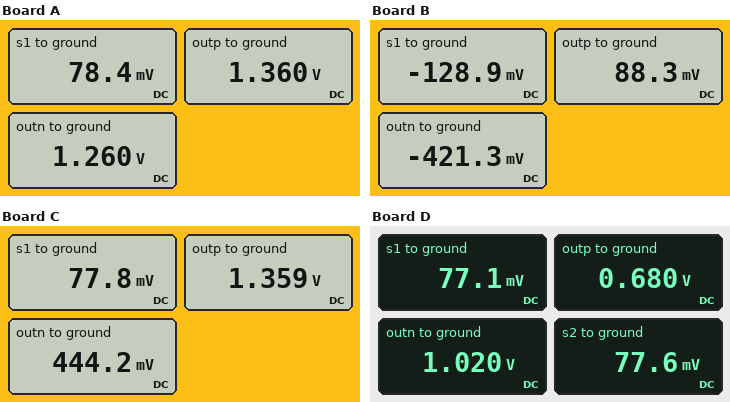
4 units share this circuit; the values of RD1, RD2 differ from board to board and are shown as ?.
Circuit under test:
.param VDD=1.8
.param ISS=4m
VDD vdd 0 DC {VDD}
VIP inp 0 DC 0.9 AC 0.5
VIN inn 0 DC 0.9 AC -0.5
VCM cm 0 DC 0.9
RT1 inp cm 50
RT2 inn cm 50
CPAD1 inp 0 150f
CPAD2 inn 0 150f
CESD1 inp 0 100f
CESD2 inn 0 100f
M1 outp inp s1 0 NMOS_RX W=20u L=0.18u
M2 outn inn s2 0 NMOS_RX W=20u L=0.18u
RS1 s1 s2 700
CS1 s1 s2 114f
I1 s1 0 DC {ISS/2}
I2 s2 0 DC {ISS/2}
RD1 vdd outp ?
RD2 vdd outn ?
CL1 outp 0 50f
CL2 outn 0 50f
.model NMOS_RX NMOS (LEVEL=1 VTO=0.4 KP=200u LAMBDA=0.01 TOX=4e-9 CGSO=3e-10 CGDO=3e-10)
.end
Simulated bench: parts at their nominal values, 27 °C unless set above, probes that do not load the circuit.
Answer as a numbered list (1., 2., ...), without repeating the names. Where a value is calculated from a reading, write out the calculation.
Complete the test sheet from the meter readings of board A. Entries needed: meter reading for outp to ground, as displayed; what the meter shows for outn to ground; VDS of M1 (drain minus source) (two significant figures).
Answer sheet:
1. 1.360 V
2. 1.260 V
3. 1.36 V - 78.4 mV = 1.3 V
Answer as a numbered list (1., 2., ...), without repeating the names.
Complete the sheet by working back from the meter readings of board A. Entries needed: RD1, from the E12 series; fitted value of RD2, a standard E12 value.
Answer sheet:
1. 220 Ω
2. 270 Ω
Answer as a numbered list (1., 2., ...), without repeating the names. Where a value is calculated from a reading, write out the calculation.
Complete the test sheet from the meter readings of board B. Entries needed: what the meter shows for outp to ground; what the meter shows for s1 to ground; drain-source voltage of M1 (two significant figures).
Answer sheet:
1. 88.3 mV
2. -128.9 mV
3. 88.3 mV - (-128.9 mV) = 220 mV
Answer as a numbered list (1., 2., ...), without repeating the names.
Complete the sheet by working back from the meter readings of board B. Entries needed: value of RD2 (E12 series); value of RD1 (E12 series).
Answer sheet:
1. 1.5 kΩ
2. 680 Ω
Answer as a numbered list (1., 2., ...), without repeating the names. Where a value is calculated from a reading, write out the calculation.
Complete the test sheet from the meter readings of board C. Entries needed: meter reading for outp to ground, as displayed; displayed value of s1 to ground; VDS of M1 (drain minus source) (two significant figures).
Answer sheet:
1. 1.359 V
2. 77.8 mV
3. 1.359 V - 77.8 mV = 1.3 V
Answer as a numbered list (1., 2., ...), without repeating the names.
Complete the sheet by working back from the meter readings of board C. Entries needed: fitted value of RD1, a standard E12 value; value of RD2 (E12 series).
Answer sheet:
1. 220 Ω
2. 680 Ω
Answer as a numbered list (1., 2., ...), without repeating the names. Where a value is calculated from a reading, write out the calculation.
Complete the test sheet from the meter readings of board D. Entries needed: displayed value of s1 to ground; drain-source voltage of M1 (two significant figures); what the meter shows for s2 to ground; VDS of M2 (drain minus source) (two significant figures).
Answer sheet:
1. 77.1 mV
2. 680 mV - 77.1 mV = 600 mV
3. 77.6 mV
4. 1.02 V - 77.6 mV = 940 mV
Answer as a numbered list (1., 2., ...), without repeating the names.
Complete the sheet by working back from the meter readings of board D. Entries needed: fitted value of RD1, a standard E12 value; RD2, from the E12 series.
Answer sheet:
1. 560 Ω
2. 390 Ω
